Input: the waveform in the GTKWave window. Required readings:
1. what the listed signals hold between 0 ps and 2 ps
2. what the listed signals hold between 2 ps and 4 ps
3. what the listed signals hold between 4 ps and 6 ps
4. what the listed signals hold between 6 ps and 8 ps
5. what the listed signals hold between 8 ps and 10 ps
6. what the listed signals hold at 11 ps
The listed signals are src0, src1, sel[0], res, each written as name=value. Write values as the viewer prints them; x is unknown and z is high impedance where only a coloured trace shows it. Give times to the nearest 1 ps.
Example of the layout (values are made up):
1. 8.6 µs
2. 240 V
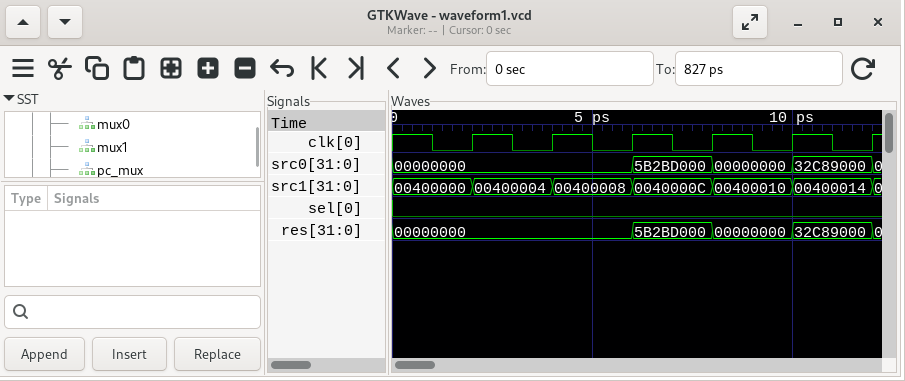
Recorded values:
1. src0=00000000, src1=00400000, sel[0]=0, res=00000000
2. src0=00000000, src1=00400004, sel[0]=0, res=00000000
3. src0=00000000, src1=00400008, sel[0]=0, res=00000000
4. src0=5B2BD000, src1=0040000C, sel[0]=0, res=5B2BD000
5. src0=00000000, src1=00400010, sel[0]=0, res=00000000
6. src0=32C89000, src1=00400014, sel[0]=0, res=32C89000
